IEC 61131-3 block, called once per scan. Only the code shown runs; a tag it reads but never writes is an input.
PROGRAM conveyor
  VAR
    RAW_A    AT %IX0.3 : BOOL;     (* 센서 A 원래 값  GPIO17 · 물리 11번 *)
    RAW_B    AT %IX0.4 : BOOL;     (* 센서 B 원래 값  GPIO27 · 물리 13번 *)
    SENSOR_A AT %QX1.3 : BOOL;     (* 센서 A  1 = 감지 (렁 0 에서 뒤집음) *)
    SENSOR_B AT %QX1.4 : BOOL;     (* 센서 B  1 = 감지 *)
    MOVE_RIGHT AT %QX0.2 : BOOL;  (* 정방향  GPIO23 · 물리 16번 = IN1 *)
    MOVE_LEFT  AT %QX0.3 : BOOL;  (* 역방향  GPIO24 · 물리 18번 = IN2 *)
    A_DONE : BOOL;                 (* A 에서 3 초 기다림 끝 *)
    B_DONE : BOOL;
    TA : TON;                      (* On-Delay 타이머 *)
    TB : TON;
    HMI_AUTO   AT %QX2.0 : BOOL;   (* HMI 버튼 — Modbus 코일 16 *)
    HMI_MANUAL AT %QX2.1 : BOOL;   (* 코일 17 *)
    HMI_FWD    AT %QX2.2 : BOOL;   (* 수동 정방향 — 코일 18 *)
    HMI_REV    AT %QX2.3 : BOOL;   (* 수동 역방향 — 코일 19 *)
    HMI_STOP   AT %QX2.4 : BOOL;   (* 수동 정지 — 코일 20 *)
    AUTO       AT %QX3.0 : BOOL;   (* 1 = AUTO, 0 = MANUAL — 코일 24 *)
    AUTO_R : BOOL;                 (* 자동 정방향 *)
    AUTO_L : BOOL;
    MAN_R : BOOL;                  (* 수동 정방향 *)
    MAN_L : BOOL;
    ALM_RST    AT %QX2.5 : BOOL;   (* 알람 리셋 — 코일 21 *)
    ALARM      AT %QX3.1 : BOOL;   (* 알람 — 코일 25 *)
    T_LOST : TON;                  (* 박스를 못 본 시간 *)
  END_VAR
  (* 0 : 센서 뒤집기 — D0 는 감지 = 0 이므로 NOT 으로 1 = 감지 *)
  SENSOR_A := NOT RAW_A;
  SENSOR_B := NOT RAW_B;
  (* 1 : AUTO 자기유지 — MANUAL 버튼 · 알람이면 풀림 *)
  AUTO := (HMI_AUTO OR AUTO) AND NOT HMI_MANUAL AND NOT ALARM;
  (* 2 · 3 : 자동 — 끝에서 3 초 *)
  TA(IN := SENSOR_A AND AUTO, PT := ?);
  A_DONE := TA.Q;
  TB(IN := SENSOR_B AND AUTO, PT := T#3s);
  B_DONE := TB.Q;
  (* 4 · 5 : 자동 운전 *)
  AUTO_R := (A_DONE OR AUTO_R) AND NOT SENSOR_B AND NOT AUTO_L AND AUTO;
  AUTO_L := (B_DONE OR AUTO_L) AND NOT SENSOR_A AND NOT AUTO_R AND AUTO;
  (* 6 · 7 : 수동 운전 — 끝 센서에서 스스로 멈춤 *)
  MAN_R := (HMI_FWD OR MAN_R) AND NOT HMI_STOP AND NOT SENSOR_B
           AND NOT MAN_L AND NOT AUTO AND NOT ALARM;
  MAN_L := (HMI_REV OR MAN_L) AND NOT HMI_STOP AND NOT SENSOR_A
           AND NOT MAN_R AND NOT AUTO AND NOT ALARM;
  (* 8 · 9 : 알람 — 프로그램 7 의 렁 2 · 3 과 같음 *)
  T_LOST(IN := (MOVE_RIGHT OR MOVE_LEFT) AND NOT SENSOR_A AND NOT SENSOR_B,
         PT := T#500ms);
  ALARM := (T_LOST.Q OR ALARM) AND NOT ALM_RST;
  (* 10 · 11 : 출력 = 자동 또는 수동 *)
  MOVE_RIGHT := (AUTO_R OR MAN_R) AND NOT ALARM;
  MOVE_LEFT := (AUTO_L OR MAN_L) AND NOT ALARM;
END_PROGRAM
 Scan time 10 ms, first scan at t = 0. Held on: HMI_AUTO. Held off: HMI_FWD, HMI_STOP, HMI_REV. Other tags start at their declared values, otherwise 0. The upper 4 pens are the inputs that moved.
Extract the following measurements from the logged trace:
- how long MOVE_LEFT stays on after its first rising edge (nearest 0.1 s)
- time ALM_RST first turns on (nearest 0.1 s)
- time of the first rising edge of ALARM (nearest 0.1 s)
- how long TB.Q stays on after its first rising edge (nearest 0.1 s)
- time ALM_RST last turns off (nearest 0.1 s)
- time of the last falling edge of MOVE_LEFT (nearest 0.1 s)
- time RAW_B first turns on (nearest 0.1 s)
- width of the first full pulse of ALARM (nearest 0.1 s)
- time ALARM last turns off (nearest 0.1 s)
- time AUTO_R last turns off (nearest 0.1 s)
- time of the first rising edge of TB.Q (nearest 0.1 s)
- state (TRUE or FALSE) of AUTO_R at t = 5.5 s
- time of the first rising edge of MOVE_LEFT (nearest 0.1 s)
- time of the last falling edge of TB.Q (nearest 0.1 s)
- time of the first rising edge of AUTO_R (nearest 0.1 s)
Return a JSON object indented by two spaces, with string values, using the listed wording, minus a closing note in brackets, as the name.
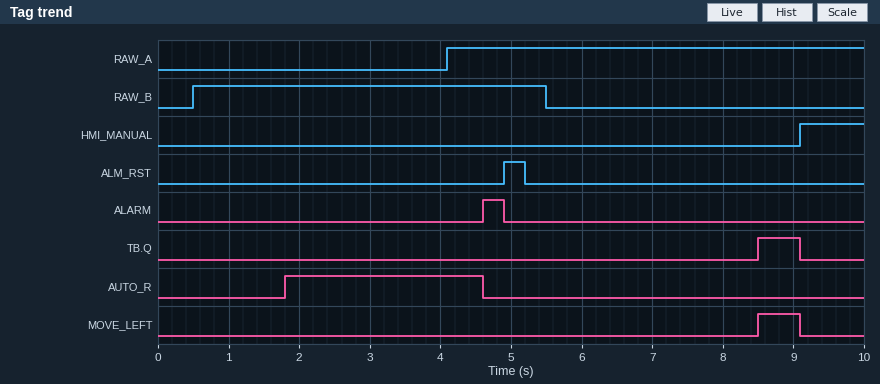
{
  "how long MOVE_LEFT stays on after its first rising edge": "0.6 s",
  "time ALM_RST first turns on": "4.9 s",
  "time of the first rising edge of ALARM": "4.6 s",
  "how long TB.Q stays on after its first rising edge": "0.6 s",
  "time ALM_RST last turns off": "5.2 s",
  "time of the last falling edge of MOVE_LEFT": "9.1 s",
  "time RAW_B first turns on": "0.5 s",
  "width of the first full pulse of ALARM": "0.3 s",
  "time ALARM last turns off": "4.9 s",
  "time AUTO_R last turns off": "4.6 s",
  "time of the first rising edge of TB.Q": "8.5 s",
  "state (TRUE or FALSE) of AUTO_R at t = 5.5 s": "FALSE",
  "time of the first rising edge of MOVE_LEFT": "8.5 s",
  "time of the last falling edge of TB.Q": "9.1 s",
  "time of the first rising edge of AUTO_R": "1.8 s"
}
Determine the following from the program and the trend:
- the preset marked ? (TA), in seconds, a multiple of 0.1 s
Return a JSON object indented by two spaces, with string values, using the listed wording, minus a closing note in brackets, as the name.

{
  "the preset marked ? (TA), in seconds, a multiple of 0.1 s": "1.8 s"
}
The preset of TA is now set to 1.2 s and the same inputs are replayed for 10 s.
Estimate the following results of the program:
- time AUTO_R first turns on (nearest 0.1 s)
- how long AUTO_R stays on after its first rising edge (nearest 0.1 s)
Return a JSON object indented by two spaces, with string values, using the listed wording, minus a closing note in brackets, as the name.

{
  "time AUTO_R first turns on": "1.2 s",
  "how long AUTO_R stays on after its first rising edge": "3.4 s"
}
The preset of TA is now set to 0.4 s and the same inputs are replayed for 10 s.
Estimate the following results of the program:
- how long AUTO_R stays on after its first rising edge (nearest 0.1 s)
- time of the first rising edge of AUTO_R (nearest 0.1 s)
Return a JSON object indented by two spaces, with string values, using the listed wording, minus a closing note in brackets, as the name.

{
  "how long AUTO_R stays on after its first rising edge": "4.1 s",
  "time of the first rising edge of AUTO_R": "0.5 s"
}
